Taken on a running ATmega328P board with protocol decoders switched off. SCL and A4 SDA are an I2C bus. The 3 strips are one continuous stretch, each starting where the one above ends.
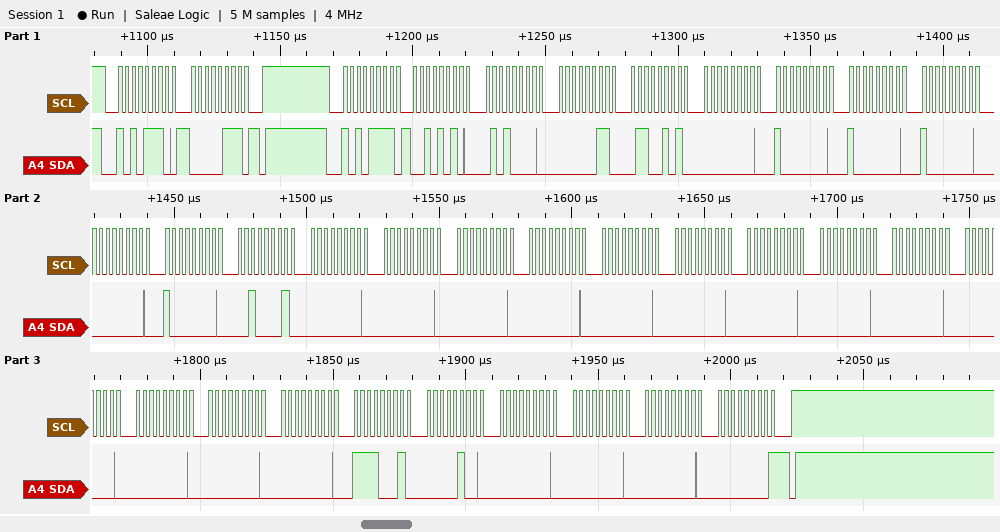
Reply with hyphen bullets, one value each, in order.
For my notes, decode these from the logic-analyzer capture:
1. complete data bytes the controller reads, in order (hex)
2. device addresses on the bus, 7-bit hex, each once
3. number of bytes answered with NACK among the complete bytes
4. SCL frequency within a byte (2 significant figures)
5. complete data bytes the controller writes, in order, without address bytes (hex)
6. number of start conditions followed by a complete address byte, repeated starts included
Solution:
- 2A 50 03 65 00 80 80 80 00 80 21 00 00 00 00 00 00 00 00 00 00 00 00 00 F1 04 00 00 00 00
- 0x57
- 1
- 400 kHz
- 07
- 2
